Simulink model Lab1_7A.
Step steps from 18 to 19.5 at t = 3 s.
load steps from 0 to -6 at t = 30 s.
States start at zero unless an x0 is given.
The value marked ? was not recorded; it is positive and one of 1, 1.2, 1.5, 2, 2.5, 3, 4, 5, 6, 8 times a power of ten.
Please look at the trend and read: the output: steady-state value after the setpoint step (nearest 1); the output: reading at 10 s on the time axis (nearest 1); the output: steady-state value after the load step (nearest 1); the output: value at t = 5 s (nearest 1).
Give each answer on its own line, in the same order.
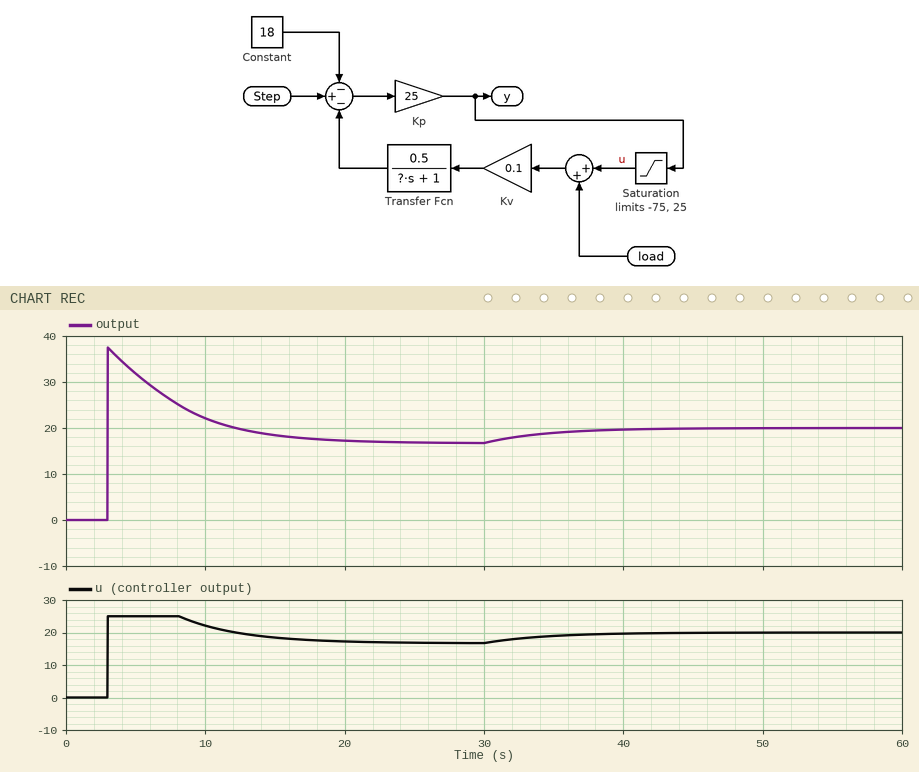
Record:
17
22
20
32
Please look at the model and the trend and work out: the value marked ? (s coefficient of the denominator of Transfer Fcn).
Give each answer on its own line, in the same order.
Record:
10
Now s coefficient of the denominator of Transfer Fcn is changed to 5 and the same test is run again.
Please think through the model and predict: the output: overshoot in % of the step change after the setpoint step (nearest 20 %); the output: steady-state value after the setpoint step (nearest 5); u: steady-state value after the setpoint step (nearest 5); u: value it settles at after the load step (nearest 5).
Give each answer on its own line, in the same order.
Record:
120 %
15
15
20
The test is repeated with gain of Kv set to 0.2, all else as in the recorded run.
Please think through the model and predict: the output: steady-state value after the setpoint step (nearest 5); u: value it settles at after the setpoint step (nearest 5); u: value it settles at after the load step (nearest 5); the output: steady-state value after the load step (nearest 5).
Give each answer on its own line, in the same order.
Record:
10
10
15
15
